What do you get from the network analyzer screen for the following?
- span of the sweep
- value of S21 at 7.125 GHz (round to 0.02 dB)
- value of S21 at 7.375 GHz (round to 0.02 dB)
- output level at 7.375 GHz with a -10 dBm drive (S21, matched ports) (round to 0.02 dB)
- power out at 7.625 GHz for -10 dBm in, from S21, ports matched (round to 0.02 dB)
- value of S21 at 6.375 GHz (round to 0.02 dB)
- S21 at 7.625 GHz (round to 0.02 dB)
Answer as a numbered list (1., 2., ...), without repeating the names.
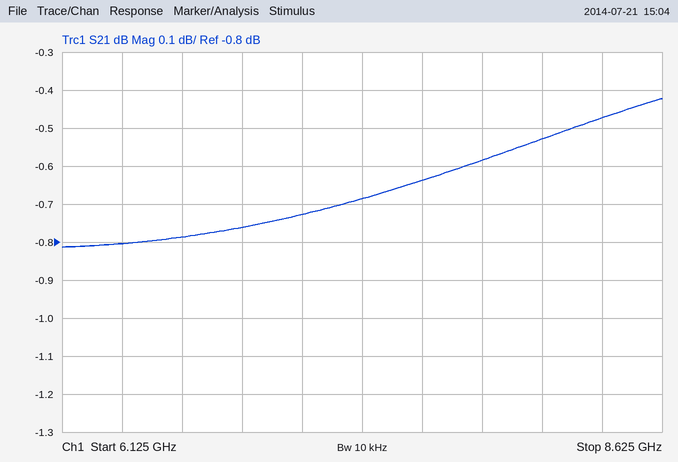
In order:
1. 2.5 GHz
2. -0.72 dB
3. -0.68 dB
4. -10.68 dBm
5. -10.64 dBm
6. -0.80 dB
7. -0.64 dB
